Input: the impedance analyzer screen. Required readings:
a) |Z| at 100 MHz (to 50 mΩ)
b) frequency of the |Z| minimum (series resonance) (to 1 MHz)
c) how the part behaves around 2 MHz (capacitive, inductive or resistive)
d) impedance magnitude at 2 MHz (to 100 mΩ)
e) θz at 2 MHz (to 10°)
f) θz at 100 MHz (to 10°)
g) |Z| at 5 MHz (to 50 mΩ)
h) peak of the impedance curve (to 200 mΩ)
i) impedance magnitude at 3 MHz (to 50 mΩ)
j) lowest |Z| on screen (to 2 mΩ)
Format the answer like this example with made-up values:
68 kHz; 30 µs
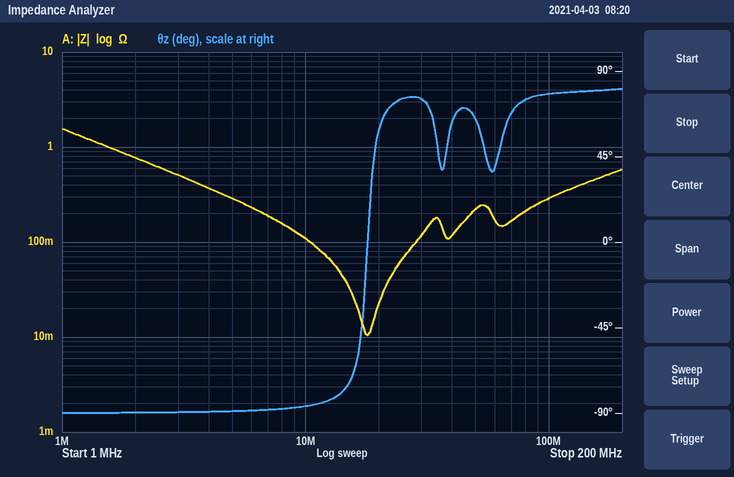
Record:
300 mΩ; 18 MHz; capacitive; 800 mΩ; -90°; 80°; 300 mΩ; 1.6 Ω; 500 mΩ; 10 mΩ
